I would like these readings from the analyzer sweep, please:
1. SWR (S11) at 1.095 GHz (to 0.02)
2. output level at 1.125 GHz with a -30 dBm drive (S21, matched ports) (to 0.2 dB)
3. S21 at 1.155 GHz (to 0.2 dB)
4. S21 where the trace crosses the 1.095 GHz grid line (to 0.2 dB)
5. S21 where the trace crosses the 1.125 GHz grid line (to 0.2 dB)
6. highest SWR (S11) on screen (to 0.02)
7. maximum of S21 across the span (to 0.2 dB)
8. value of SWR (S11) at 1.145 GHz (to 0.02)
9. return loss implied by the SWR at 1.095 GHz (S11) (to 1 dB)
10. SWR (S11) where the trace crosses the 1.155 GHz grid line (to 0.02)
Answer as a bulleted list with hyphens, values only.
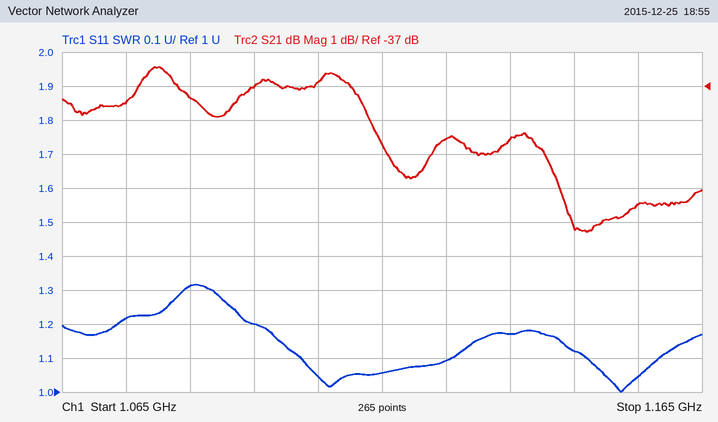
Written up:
- 1.20
- -68.6 dBm
- -40.4 dB
- -37.0 dB
- -38.6 dB
- 1.32
- -36.4 dB
- 1.12
- 21 dB
- 1.04
